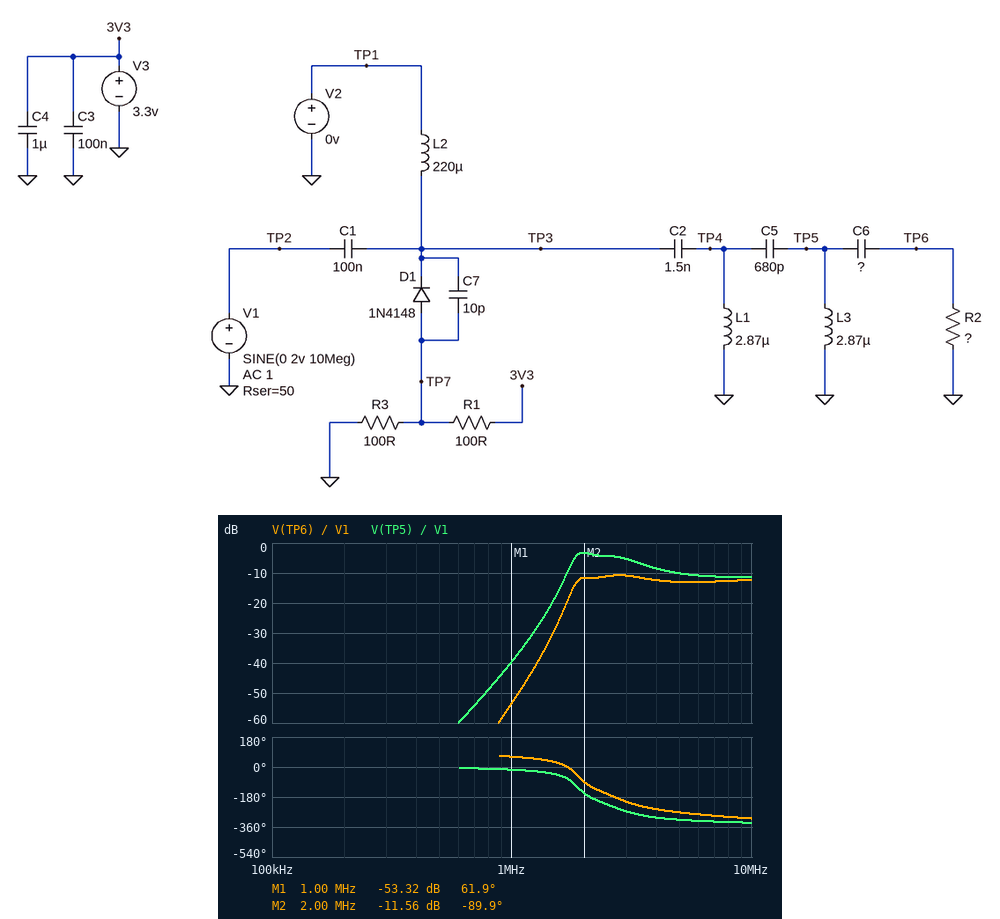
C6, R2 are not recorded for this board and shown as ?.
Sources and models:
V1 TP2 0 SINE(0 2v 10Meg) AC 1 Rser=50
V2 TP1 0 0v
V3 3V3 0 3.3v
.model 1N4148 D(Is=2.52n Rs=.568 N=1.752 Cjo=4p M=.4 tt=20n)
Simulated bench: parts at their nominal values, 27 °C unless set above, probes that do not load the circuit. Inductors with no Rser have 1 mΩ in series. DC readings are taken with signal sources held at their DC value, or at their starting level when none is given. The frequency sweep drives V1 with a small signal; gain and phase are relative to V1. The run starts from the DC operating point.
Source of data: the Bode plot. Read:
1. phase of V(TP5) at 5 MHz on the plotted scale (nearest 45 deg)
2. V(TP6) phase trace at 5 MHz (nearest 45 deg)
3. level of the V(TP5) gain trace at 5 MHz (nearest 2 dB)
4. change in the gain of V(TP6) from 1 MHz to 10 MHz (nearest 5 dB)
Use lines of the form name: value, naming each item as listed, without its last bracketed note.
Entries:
phase of V(TP5) at 5 MHz on the plotted scale: -315 deg
V(TP6) phase trace at 5 MHz: -270 deg
level of the V(TP5) gain trace at 5 MHz: -10 dB
change in the gain of V(TP6) from 1 MHz to 10 MHz: 40 dB
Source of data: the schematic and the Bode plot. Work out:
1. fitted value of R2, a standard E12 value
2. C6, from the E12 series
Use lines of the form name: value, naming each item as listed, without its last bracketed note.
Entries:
fitted value of R2, a standard E12 value: 33 Ω
C6, from the E12 series: 1 nF
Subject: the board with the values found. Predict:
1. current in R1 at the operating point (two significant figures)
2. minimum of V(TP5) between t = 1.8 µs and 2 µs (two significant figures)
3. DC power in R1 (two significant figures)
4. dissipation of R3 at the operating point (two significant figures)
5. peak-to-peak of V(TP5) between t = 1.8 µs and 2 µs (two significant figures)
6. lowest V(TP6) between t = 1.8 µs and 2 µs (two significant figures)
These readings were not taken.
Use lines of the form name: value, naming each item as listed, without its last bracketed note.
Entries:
current in R1 at the operating point: 26 mA
minimum of V(TP5) between t = 1.8 µs and 2 µs: -550 mV
DC power in R1: 66 mW
dissipation of R3 at the operating point: 5.3 mW
peak-to-peak of V(TP5) between t = 1.8 µs and 2 µs: 1.1 V
lowest V(TP6) between t = 1.8 µs and 2 µs: -490 mV
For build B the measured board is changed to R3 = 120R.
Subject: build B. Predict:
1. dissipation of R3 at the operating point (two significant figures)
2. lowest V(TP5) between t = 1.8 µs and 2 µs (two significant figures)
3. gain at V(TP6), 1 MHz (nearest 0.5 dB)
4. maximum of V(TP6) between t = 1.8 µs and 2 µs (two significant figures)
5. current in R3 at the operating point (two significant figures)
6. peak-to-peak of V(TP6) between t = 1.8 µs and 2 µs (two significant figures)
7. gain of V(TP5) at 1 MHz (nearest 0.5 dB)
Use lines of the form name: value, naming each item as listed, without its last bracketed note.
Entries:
dissipation of R3 at the operating point: 4.4 mW
lowest V(TP5) between t = 1.8 µs and 2 µs: -560 mV
gain at V(TP6), 1 MHz: -53.0 dB
maximum of V(TP6) between t = 1.8 µs and 2 µs: 500 mV
current in R3 at the operating point: 6.1 mA
peak-to-peak of V(TP6) between t = 1.8 µs and 2 µs: 1.0 V
gain of V(TP5) at 1 MHz: -39.0 dB
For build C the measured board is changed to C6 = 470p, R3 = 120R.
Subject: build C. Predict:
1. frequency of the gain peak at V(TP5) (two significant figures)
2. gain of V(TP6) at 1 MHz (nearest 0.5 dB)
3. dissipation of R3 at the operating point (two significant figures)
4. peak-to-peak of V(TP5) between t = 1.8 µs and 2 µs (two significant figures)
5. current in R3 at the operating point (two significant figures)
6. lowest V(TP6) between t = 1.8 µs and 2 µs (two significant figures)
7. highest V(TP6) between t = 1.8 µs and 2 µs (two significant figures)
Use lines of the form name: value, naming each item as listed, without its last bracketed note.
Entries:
frequency of the gain peak at V(TP5): 3.2 MHz
gain of V(TP6) at 1 MHz: -60.0 dB
dissipation of R3 at the operating point: 4.4 mW
peak-to-peak of V(TP5) between t = 1.8 µs and 2 µs: 1.3 V
current in R3 at the operating point: 6.1 mA
lowest V(TP6) between t = 1.8 µs and 2 µs: -450 mV
highest V(TP6) between t = 1.8 µs and 2 µs: 450 mV
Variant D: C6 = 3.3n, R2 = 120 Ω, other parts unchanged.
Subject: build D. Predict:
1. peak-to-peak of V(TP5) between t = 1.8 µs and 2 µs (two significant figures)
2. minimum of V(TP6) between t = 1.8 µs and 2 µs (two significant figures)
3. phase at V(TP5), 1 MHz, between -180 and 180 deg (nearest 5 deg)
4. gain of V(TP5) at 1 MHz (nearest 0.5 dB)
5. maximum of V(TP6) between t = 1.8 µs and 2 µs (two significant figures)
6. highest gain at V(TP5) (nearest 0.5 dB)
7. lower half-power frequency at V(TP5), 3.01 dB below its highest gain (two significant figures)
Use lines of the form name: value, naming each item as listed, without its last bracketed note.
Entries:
peak-to-peak of V(TP5) between t = 1.8 µs and 2 µs: 1.9 V
minimum of V(TP6) between t = 1.8 µs and 2 µs: -930 mV
phase at V(TP5), 1 MHz, between -180 and 180 deg: -25 deg
gain of V(TP5) at 1 MHz: -40.0 dB
maximum of V(TP6) between t = 1.8 µs and 2 µs: 930 mV
highest gain at V(TP5): -5.0 dB
lower half-power frequency at V(TP5), 3.01 dB below its highest gain: 1.9 MHz
